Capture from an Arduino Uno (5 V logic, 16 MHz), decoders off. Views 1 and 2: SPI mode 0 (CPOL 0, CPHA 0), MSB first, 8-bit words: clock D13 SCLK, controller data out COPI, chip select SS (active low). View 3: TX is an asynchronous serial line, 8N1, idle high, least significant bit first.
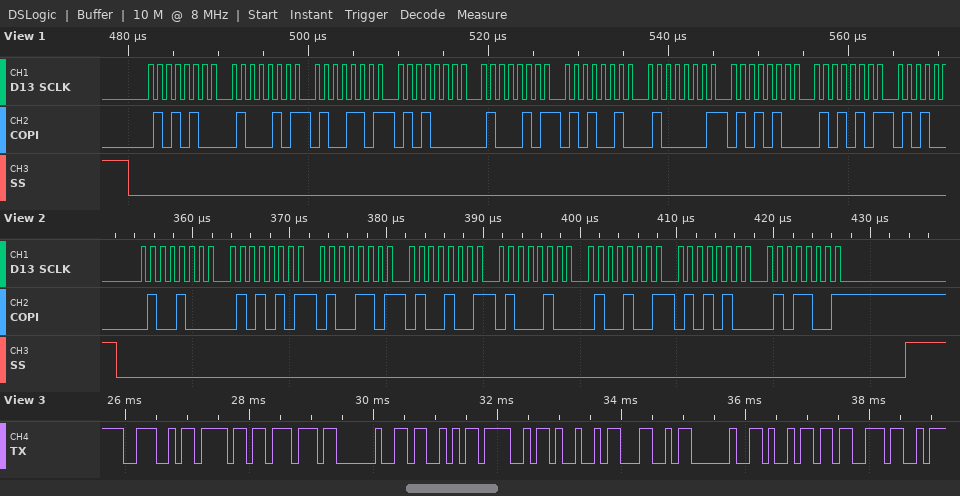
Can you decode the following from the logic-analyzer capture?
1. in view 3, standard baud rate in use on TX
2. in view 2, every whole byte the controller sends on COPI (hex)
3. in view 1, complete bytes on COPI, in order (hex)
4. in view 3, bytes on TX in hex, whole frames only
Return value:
9600 baud
48 55 4D 49 44 49 54 59
54 45 4D 50 45 52 41 54 55
4E 6F 77 20 53 4F 49 4C 20 69 73
